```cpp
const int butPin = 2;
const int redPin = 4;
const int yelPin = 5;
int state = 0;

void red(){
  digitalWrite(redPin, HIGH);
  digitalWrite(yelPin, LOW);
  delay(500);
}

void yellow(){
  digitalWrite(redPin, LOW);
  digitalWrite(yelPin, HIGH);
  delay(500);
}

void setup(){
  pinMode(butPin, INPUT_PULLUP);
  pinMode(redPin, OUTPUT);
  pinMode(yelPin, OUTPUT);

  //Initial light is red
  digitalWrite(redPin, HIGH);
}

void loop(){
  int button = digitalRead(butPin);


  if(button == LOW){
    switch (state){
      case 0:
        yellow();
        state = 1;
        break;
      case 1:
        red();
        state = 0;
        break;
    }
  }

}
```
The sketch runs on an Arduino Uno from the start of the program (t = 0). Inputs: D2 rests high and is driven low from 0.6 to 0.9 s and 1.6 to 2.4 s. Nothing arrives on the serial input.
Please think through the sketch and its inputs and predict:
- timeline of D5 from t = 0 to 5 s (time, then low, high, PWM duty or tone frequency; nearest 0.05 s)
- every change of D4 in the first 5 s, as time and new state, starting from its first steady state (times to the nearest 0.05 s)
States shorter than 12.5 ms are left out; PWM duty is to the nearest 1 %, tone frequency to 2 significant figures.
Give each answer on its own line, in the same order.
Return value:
0 s low; 0.6 s high; 1.6 s low; 2.1 s high
0 s high; 0.6 s low; 1.6 s high; 2.1 s low
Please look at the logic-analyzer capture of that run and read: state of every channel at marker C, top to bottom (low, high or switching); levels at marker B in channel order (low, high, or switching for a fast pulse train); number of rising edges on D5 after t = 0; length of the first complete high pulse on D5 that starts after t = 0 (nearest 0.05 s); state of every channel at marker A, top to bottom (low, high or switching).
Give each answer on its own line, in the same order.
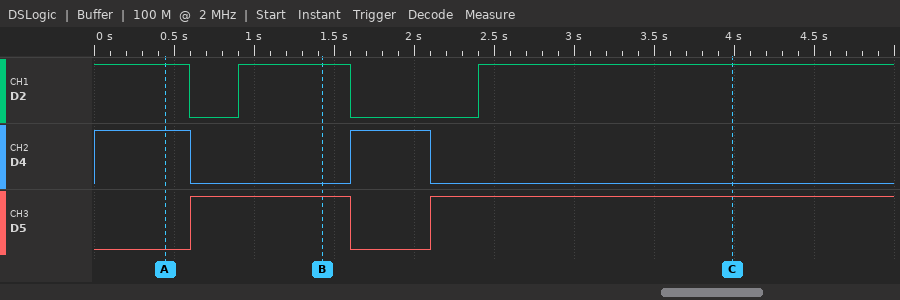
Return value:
D2 high, D4 low, D5 high
D2 high, D4 low, D5 high
2
1.00 s
D2 high, D4 high, D5 low
